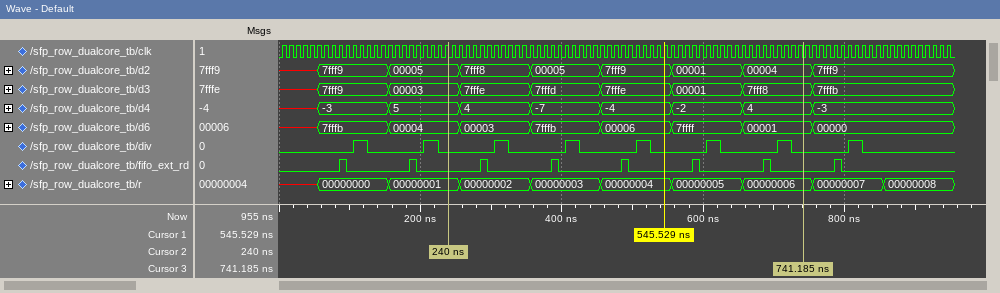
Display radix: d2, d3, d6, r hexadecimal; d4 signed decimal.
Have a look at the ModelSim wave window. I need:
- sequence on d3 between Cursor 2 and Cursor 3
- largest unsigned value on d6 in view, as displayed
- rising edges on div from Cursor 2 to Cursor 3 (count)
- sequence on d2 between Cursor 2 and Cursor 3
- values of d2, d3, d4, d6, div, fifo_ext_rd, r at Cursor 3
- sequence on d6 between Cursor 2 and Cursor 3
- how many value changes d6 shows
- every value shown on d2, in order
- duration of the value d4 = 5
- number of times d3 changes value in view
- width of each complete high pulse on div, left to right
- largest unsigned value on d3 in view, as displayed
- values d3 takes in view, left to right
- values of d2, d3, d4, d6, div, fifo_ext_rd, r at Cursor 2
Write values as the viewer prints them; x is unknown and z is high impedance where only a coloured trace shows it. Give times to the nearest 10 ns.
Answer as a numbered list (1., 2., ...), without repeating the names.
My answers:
1. 00003, 7fffe, 7fffd, 7fffe, 00001, 7fff8
2. 7ffff
3. 5
4. 00005, 7fff8, 00005, 7fff9, 00001, 00004
5. d2=00004, d3=7fff8, d4=4, d6=00001, div=0, fifo_ext_rd=0, r=00000006
6. 00004, 00003, 7fffb, 00006, 7ffff, 00001
7. 8
8. x, 7fff9, 00005, 7fff8, 00005, 7fff9, 00001, 00004, 7fff9
9. 100 ns
10. 8
11. 20 ns, 20 ns, 20 ns, 20 ns, 20 ns, 20 ns, 20 ns, 20 ns
12. 7fffe
13. x, 7fff9, 00003, 7fffe, 7fffd, 7fffe, 00001, 7fff8, 7fffb
14. d2=00005, d3=00003, d4=5, d6=00004, div=0, fifo_ext_rd=0, r=00000001
